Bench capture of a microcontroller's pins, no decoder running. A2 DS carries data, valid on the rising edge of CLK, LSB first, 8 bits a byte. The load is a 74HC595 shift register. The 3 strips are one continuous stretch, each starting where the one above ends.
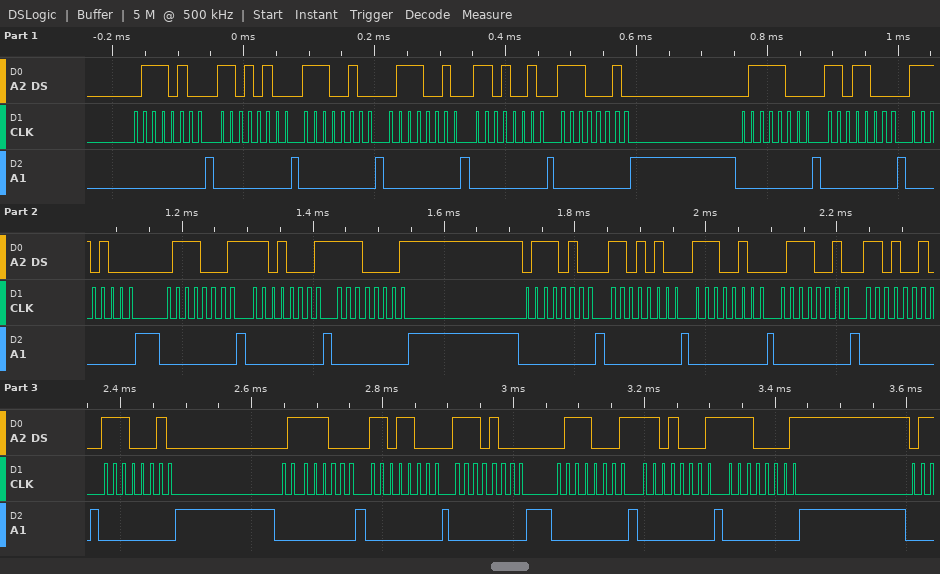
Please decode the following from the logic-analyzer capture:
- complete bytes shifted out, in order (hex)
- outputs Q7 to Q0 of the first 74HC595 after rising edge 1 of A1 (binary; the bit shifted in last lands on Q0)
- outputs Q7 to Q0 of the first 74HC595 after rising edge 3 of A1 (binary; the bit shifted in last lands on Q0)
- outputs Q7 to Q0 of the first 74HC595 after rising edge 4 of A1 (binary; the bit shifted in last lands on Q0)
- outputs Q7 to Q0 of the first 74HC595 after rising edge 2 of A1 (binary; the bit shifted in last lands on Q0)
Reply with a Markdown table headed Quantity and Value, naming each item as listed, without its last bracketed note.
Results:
| Quantity | Value |
|---|---|
| complete bytes shifted out, in order | 2E 2B 27 4E 4B 47 1E 1B 17 8E 8B 87 2E 2B 27 4E 4B 47 1E 1B 17 8E 8B 87 |
| outputs Q7 to Q0 of the first 74HC595 after rising edge 1 of A1 | 01110100 |
| outputs Q7 to Q0 of the first 74HC595 after rising edge 3 of A1 | 11100100 |
| outputs Q7 to Q0 of the first 74HC595 after rising edge 4 of A1 | 01110010 |
| outputs Q7 to Q0 of the first 74HC595 after rising edge 2 of A1 | 11010100 |
